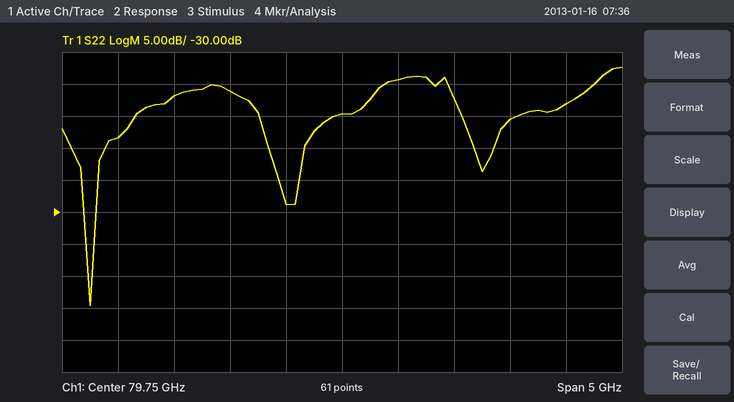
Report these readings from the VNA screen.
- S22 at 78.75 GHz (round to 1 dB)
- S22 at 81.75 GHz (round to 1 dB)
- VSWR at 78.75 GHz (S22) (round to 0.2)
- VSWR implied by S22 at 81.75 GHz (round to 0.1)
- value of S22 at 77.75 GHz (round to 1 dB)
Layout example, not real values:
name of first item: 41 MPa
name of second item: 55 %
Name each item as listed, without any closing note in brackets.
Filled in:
S22 at 78.75 GHz: -11 dB
S22 at 81.75 GHz: -13 dB
VSWR at 78.75 GHz (S22): 1.8
VSWR implied by S22 at 81.75 GHz: 1.6
value of S22 at 77.75 GHz: -18 dB
